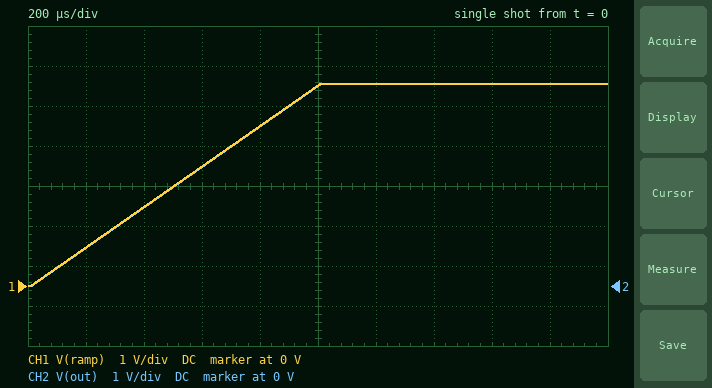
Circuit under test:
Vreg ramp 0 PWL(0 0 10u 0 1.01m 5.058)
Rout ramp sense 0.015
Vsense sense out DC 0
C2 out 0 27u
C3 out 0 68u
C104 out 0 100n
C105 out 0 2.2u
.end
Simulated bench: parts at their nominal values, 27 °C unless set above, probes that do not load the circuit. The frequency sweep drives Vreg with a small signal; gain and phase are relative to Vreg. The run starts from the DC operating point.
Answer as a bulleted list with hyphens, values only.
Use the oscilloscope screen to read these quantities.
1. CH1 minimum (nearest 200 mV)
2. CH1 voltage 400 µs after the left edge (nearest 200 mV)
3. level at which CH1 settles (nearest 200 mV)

- 0 V
- 2.0 V
- 5.0 V
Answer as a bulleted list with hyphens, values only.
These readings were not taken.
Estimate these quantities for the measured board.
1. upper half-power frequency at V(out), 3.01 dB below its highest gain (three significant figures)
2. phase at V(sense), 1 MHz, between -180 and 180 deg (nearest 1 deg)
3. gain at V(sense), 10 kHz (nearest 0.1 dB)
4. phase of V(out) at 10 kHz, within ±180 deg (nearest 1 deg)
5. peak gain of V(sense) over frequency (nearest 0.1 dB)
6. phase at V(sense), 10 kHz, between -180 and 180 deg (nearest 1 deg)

- 109 kHz
- -84 deg
- 0 dB
- -5 deg
- 0 dB
- -5 deg
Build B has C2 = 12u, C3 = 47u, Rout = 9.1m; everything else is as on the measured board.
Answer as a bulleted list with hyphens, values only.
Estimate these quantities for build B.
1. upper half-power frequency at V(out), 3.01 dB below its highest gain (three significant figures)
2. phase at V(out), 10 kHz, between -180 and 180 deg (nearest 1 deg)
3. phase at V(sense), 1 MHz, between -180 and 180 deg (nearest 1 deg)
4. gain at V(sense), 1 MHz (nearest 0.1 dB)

- 285 kHz
- -2 deg
- -74 deg
- -11.2 dB
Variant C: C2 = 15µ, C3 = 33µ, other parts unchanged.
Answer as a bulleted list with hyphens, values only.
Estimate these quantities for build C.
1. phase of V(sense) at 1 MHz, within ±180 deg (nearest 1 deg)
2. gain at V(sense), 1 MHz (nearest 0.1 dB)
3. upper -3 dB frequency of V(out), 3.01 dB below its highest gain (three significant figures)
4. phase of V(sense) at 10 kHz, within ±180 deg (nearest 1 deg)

- -78 deg
- -13.7 dB
- 211 kHz
- -3 deg
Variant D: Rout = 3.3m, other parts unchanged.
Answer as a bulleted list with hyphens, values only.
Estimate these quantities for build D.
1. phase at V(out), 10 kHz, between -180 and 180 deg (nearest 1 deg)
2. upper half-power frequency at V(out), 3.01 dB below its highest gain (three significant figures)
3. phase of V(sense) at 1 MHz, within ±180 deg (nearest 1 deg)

- -1 deg
- 496 kHz
- -64 deg
